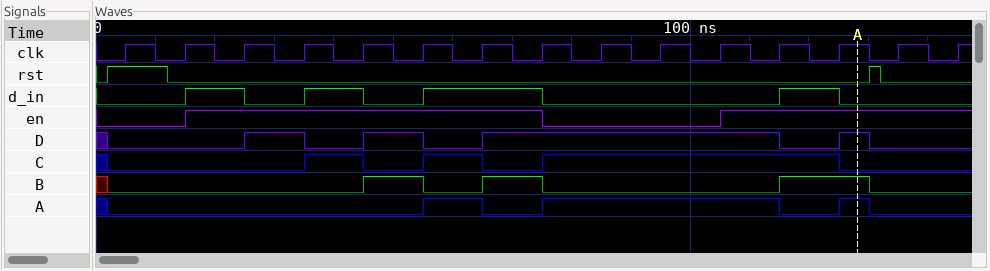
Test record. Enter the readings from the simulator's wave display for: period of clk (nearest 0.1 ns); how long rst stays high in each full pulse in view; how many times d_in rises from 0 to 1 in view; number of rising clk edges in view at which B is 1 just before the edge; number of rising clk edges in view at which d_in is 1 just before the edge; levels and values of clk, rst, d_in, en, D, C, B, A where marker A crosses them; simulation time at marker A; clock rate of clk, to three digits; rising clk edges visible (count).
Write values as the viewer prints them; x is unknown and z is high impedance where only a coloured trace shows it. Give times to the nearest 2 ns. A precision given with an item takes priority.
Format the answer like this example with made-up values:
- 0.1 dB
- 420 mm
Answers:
- 10 ns
- 10 ns, 2 ns
- 4
- 3
- 5
- clk=1, rst=0, d_in=0, en=1, D=1, C=0, B=1, A=1
- 128 ns
- 100 MHz
- 15
